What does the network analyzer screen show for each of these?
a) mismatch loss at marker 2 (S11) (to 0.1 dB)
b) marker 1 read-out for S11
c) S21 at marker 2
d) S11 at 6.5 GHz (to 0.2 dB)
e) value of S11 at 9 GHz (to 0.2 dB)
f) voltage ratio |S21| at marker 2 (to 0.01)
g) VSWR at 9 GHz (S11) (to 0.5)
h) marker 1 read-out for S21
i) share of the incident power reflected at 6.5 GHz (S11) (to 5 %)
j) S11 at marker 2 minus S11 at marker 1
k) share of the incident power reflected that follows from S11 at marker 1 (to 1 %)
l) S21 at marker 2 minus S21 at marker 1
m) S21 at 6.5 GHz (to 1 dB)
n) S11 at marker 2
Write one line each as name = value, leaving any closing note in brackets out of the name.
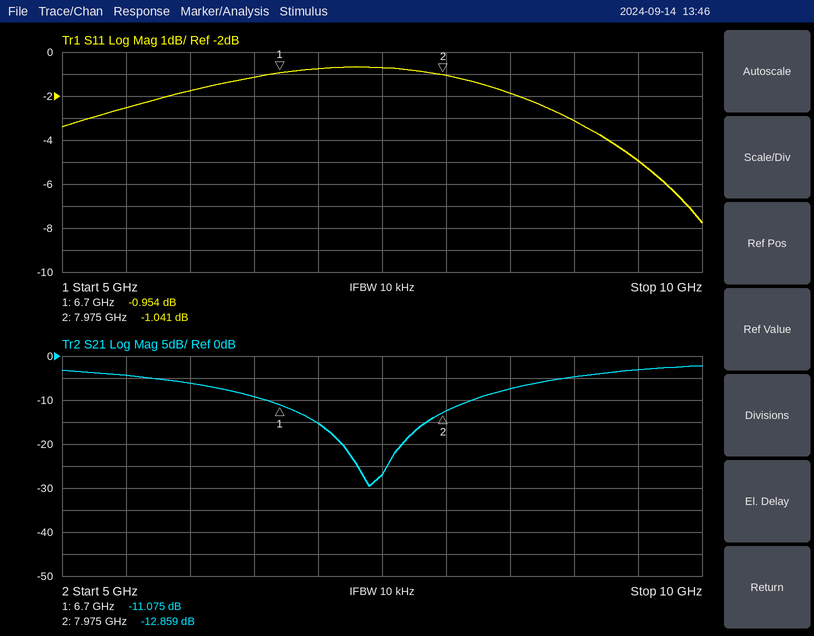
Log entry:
mismatch loss at marker 2 (S11) = 6.7 dB
marker 1 read-out for S11 = -0.954 dB
S21 at marker 2 = -12.859 dB
S11 at 6.5 GHz = -1.2 dB
value of S11 at 9 GHz = -3.2 dB
voltage ratio |S21| at marker 2 = 0.23
VSWR at 9 GHz (S11) = 5.5
marker 1 read-out for S21 = -11.075 dB
share of the incident power reflected at 6.5 GHz (S11) = 75 %
S11 at marker 2 minus S11 at marker 1 = -0.087 dB
share of the incident power reflected that follows from S11 at marker 1 = 80 %
S21 at marker 2 minus S21 at marker 1 = -1.784 dB
S21 at 6.5 GHz = -9 dB
S11 at marker 2 = -1.041 dB
